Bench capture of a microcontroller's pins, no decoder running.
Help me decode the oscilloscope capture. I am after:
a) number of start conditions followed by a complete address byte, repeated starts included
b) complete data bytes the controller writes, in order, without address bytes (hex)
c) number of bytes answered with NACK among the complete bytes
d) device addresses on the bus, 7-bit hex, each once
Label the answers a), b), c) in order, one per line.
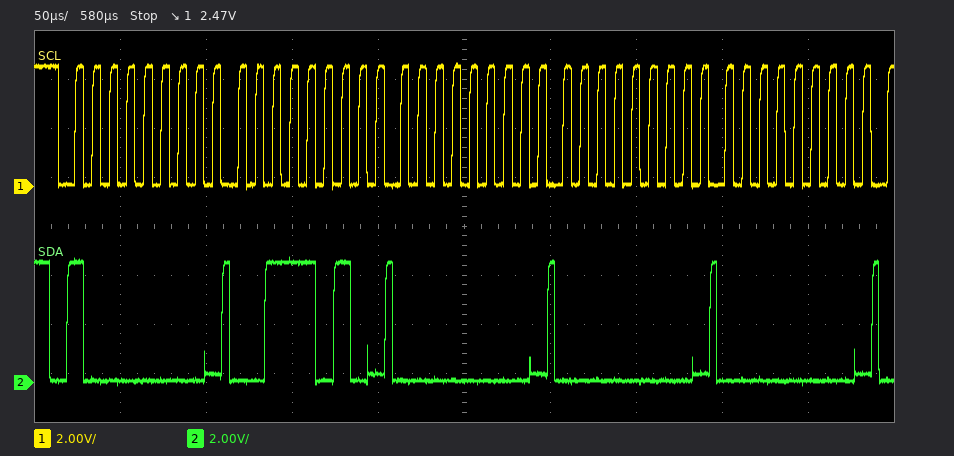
a) 1
b) 3A 00 00 00
c) 0
d) 0x40
